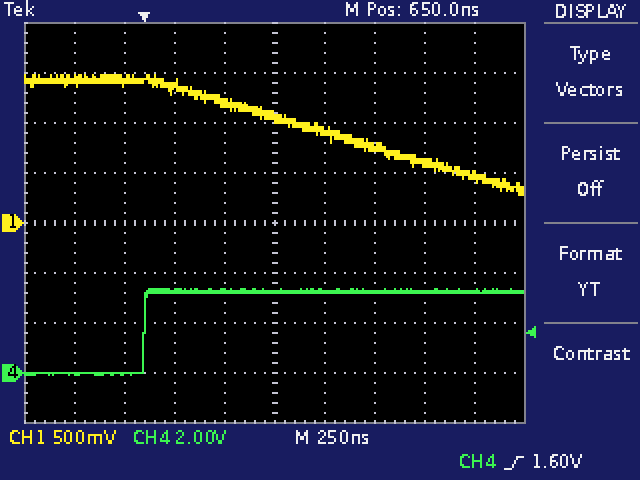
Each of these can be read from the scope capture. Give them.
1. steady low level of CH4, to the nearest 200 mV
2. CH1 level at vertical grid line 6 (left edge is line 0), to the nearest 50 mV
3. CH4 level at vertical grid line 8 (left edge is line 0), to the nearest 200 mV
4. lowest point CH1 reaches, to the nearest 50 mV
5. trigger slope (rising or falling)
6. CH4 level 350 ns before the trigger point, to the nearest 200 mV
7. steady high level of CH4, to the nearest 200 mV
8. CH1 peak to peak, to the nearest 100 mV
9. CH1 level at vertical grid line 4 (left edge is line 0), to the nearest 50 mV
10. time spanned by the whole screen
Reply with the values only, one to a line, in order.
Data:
0.0 V
900 mV
3.2 V
300 mV
rising
0.0 V
3.2 V
1.20 V
1.20 V
2.5 µs
